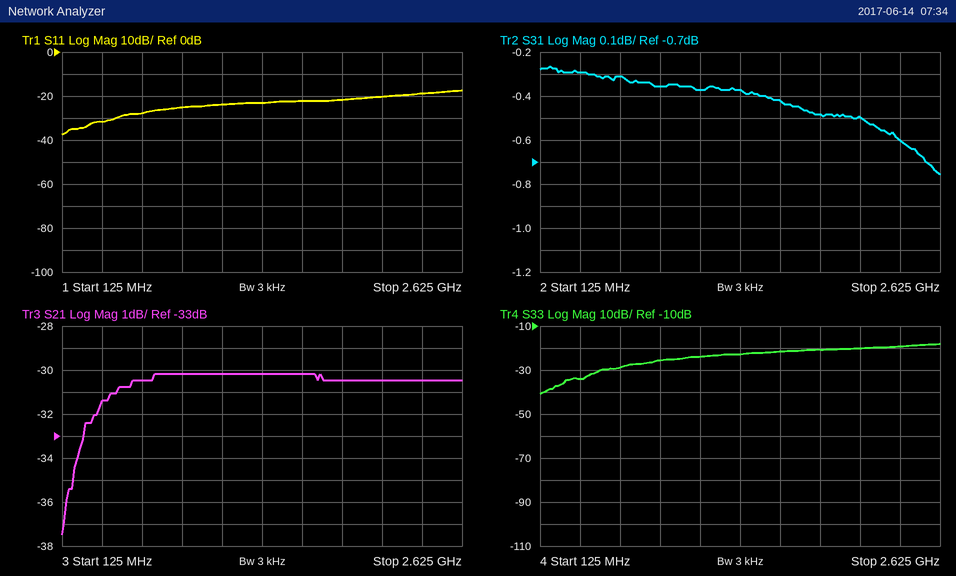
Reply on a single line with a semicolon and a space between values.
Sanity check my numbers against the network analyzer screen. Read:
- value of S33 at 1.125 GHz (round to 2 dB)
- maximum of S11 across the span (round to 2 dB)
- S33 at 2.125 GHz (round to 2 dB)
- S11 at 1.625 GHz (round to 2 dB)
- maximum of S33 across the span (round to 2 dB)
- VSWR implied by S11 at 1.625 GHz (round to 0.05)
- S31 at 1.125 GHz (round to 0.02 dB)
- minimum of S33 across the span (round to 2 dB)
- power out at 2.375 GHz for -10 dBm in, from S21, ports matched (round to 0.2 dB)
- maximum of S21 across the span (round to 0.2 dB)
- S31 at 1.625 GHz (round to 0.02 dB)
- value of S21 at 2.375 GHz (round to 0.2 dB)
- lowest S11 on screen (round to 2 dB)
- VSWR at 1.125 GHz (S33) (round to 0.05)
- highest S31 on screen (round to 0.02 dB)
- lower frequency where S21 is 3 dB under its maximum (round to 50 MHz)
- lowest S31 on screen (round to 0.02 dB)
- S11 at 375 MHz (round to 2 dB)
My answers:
-24 dB; -18 dB; -20 dB; -22 dB; -18 dB; 1.15; -0.38 dB; -40 dB; -40.4 dBm; -30.2 dB; -0.42 dB; -30.4 dB; -38 dB; 1.15; -0.26 dB; 250 MHz; -0.76 dB; -32 dB
